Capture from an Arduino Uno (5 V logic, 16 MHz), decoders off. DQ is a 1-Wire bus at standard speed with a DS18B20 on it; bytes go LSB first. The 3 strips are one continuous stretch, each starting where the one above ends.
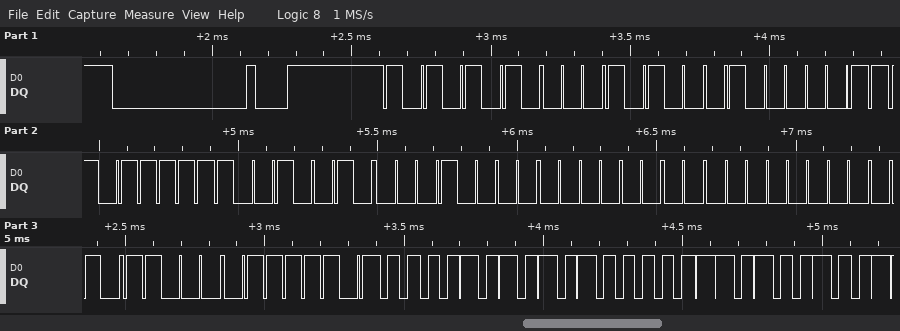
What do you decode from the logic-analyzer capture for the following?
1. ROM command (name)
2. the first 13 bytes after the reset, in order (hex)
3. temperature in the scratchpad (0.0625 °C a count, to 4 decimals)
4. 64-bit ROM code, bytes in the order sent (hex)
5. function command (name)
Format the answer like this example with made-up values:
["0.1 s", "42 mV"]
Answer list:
["Match ROM", "55 28 82 FB 49 08 00 00 1A BE 50 05 4B", "85.0000 °C", "28 82 FB 49 08 00 00 1A", "Read Scratchpad"]
